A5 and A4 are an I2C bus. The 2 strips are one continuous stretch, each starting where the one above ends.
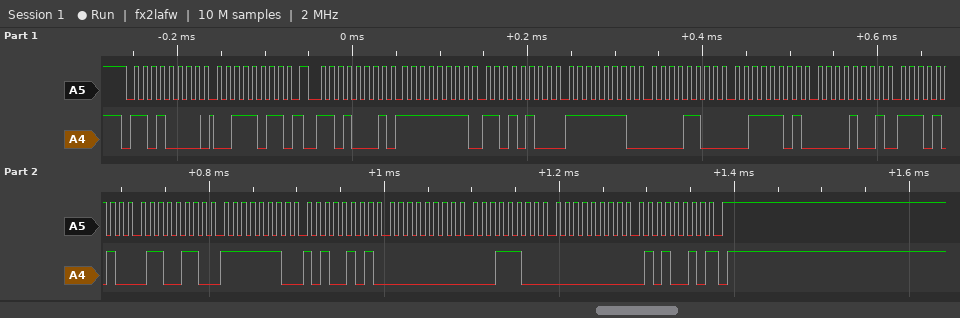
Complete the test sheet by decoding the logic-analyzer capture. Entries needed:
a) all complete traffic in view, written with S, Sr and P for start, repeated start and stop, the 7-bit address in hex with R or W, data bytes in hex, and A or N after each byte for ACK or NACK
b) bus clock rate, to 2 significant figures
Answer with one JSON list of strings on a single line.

["S 68W A 3B A Sr 68R A FF A D4 A FE A 0C A 3D A 09 A EA A 66 A FE A A5 A 00 A 1C A 00 A 52 N P", "100 kHz"]
